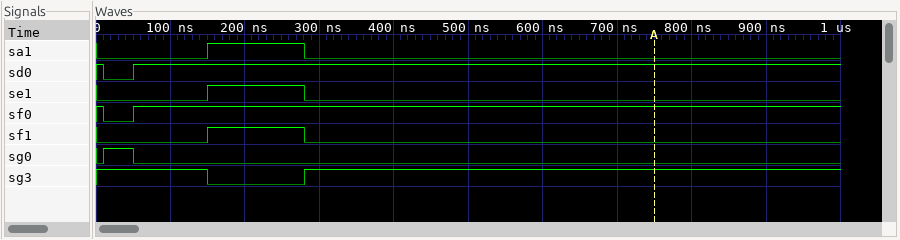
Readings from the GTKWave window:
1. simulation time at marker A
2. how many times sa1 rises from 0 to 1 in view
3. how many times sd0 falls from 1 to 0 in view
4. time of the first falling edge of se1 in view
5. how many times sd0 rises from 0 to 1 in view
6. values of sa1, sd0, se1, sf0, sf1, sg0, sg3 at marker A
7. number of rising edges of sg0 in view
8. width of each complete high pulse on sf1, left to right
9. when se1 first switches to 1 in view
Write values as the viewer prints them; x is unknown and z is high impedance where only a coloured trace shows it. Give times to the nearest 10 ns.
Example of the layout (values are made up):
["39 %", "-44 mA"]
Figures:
["750 ns", "1", "1", "280 ns", "1", "sa1=0, sd0=1, se1=0, sf0=1, sf1=0, sg0=0, sg3=1", "1", "130 ns", "150 ns"]
